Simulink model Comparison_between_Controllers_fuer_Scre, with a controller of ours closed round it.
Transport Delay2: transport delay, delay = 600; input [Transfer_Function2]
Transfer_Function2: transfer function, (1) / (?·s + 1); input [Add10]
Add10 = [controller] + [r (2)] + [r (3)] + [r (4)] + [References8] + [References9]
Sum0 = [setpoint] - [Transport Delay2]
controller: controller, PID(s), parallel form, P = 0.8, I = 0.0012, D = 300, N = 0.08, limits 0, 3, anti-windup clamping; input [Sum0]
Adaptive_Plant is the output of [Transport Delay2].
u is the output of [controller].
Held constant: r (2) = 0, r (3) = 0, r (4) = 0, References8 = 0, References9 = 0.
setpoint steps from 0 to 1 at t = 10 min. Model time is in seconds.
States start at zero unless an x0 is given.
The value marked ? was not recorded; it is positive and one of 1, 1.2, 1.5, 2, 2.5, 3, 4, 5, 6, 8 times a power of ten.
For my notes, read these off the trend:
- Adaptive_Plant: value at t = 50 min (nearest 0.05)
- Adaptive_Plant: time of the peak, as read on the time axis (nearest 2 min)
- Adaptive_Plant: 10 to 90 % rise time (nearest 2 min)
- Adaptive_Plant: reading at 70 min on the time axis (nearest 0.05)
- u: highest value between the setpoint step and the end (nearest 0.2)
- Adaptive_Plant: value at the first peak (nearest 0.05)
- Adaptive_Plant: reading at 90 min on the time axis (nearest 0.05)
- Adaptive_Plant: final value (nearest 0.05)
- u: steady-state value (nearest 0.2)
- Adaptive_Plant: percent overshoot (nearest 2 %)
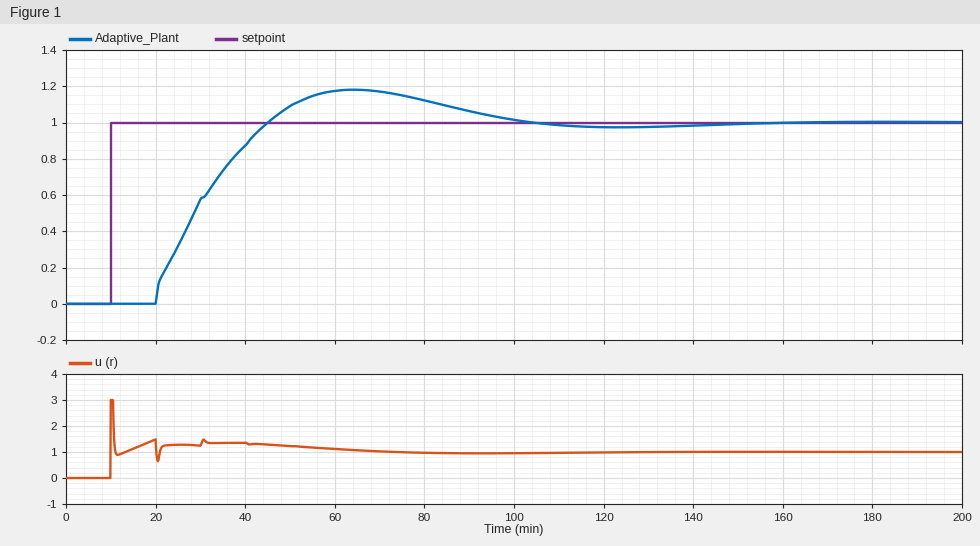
1.10
64 min
20 min
1.15
3.0
1.20
1.05
1.00
1.0
18 %
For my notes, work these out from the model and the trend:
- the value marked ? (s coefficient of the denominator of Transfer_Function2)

1000
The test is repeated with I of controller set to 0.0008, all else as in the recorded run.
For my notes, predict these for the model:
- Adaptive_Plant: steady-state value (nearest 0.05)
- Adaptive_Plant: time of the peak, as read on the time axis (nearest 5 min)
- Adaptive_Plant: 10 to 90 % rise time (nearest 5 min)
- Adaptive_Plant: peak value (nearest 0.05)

1.00
85 min
30 min
1.05
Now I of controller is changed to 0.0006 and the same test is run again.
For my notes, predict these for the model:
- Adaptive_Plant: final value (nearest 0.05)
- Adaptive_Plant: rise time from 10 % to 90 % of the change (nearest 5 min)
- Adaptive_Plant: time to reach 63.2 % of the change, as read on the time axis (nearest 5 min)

1.00
45 min
40 min
